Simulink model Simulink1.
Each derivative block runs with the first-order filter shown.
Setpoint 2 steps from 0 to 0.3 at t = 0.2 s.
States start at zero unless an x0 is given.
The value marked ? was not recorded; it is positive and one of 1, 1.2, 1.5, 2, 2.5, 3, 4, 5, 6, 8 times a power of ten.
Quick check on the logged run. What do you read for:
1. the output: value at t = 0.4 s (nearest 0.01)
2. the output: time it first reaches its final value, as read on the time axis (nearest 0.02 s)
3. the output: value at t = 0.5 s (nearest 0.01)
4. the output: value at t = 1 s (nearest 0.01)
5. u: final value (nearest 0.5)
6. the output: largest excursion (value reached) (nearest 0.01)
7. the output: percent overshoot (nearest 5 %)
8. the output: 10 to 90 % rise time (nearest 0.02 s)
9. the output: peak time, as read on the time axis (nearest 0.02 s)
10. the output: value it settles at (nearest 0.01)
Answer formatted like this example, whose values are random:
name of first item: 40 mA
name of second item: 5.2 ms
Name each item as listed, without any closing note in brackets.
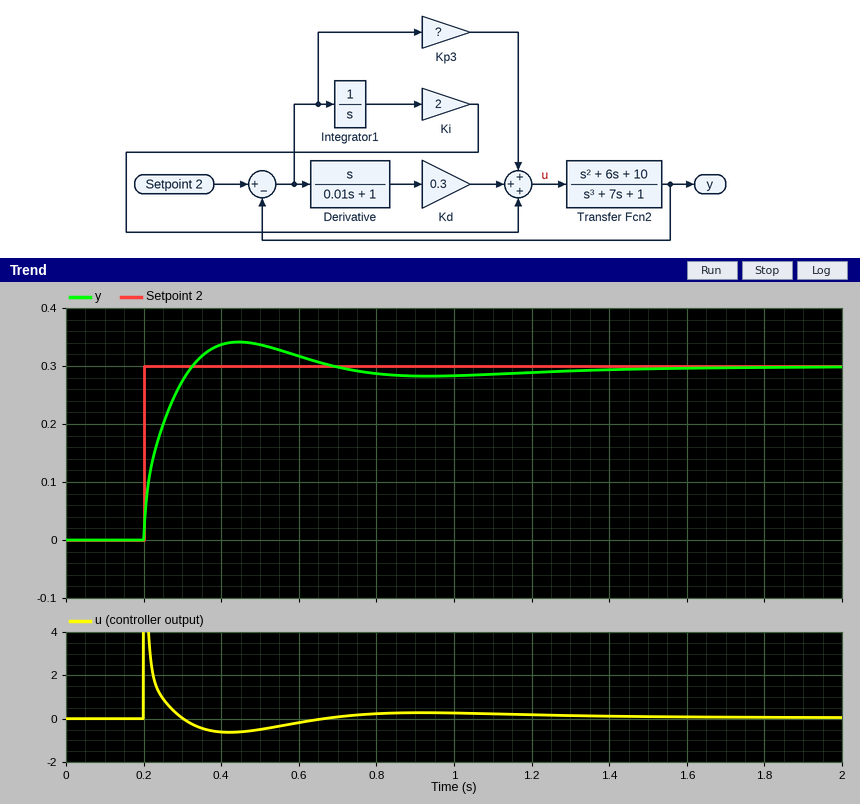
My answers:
the output: value at t = 0.4 s: 0.34
the output: time it first reaches its final value, as read on the time axis: 0.32 s
the output: value at t = 0.5 s: 0.34
the output: value at t = 1 s: 0.28
u: final value: 0.0
the output: largest excursion (value reached): 0.34
the output: percent overshoot: 15 %
the output: 10 to 90 % rise time: 0.10 s
the output: peak time, as read on the time axis: 0.44 s
the output: value it settles at: 0.30
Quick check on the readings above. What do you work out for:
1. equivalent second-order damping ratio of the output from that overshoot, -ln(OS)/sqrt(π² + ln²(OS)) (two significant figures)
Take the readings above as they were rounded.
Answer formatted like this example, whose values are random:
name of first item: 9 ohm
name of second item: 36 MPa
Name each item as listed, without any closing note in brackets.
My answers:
equivalent second-order damping ratio of the output from that overshoot, -ln(OS)/sqrt(π² + ln²(OS)): 0.52
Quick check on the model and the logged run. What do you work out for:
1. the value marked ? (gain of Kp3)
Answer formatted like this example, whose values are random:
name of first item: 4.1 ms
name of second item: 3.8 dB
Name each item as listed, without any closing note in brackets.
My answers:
the value marked ?: 15
